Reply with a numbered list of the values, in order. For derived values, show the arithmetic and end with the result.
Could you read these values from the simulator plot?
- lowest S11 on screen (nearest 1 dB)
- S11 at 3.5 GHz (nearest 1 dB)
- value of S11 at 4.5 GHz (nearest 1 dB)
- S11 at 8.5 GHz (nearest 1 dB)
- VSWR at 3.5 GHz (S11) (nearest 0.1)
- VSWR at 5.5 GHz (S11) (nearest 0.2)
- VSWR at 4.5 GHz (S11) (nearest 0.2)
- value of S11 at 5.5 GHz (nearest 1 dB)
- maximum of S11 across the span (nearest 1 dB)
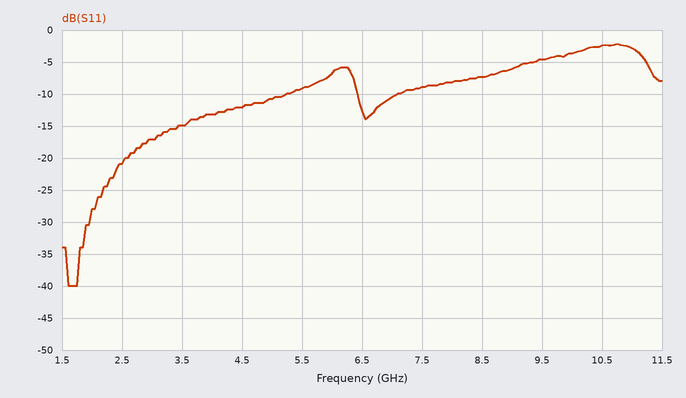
1. -40 dB
2. -15 dB
3. -12 dB
4. -7 dB
5. |Γ| = 10^(-15/20) = 0.1778; VSWR = (1 + 0.1778)/(1 − 0.1778) ≈ 1.4
6. |Γ| = 10^(-9/20) = 0.3548; VSWR = (1 + 0.3548)/(1 − 0.3548) ≈ 2.10, so 2.0 to the nearest 0.2
7. |Γ| = 10^(-12/20) = 0.2512; VSWR = (1 + 0.2512)/(1 − 0.2512) ≈ 1.67, so 1.6 to the nearest 0.2
8. -9 dB
9. -2 dB
